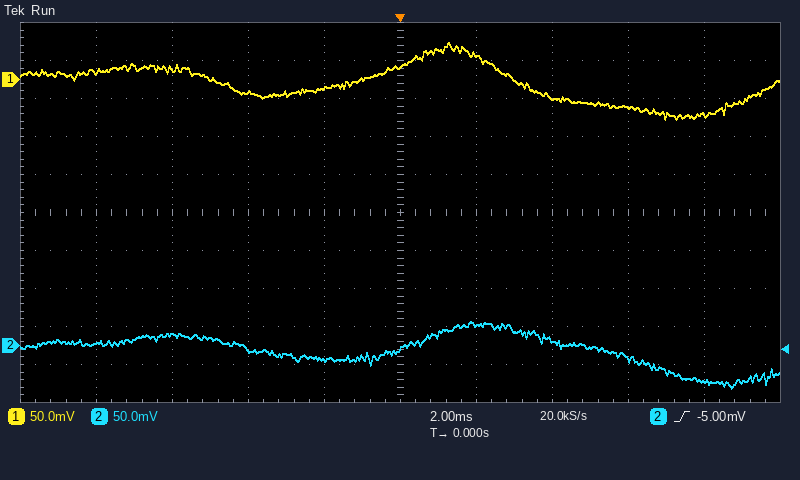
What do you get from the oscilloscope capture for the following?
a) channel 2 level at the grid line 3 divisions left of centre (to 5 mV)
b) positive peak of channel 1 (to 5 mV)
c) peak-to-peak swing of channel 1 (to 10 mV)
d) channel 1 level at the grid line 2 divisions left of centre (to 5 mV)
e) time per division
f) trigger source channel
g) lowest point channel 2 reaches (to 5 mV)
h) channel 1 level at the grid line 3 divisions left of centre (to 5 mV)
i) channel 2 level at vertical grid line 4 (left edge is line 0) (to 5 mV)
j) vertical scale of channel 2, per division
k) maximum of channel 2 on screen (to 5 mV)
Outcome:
15 mV
50 mV
100 mV
-15 mV
2 ms
channel 2
-55 mV
15 mV
-20 mV
50 mV
30 mV
